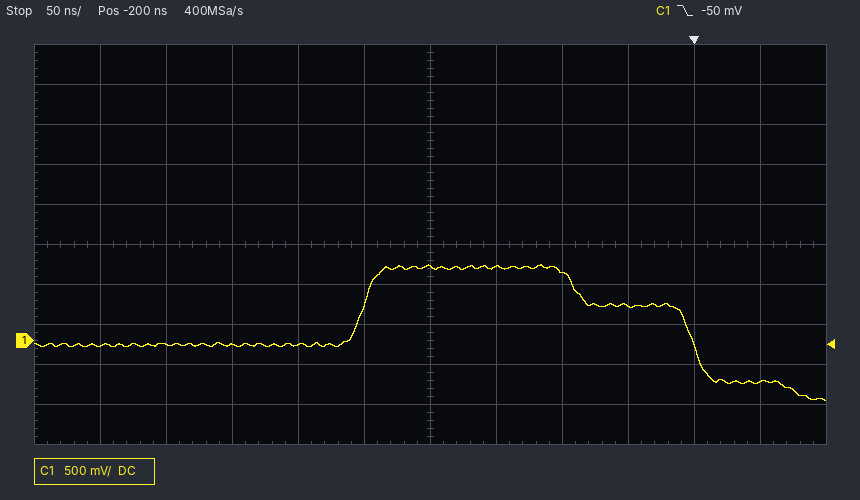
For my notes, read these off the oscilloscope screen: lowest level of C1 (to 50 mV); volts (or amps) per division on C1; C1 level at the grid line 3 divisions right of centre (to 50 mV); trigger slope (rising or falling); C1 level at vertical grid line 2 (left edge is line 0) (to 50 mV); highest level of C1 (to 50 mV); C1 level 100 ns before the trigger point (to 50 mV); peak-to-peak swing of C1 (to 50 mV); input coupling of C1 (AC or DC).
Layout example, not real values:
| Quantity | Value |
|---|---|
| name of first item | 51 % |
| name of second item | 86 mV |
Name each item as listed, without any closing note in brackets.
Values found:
| Quantity | Value |
|---|---|
| lowest level of C1 | -750 mV |
| volts (or amps) per division on C1 | 500 mV |
| C1 level at the grid line 3 divisions right of centre | 450 mV |
| trigger slope | falling |
| C1 level at vertical grid line 2 (left edge is line 0) | -50 mV |
| highest level of C1 | 950 mV |
| C1 level 100 ns before the trigger point | 850 mV |
| peak-to-peak swing of C1 | 1.70 V |
| input coupling of C1 | DC |
